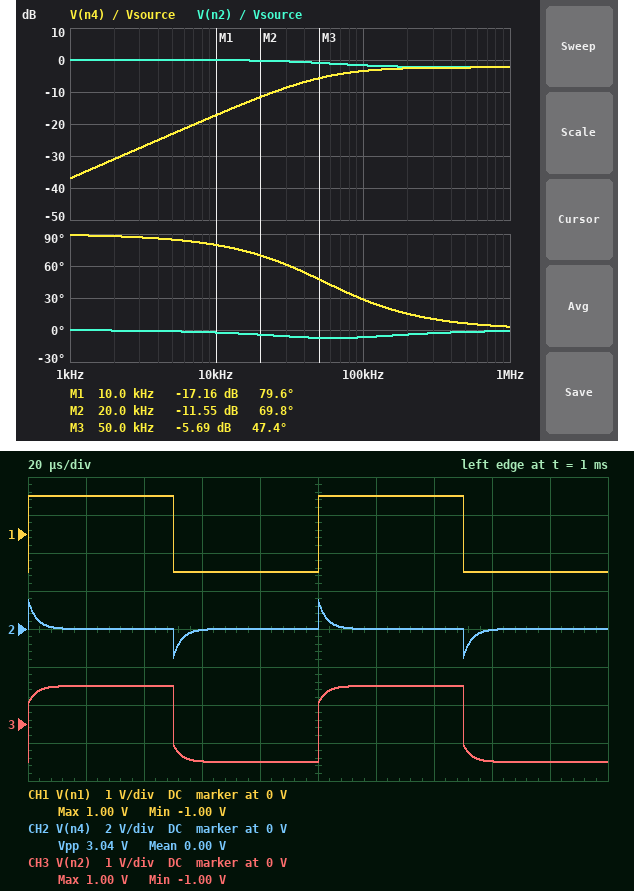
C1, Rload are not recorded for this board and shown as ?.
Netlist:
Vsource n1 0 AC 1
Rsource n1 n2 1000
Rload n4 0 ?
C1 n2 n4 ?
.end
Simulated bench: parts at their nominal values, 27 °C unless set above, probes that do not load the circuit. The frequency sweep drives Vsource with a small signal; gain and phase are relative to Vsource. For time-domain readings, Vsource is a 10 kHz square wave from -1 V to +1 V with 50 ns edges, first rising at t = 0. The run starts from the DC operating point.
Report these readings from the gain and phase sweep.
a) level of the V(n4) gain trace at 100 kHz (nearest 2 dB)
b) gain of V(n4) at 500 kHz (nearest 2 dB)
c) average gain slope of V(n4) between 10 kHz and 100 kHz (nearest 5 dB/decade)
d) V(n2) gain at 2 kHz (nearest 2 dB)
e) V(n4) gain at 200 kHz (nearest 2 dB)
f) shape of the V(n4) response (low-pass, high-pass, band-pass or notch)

-4 dB
-2 dB
15 dB/decade
0 dB
-2 dB
high-pass
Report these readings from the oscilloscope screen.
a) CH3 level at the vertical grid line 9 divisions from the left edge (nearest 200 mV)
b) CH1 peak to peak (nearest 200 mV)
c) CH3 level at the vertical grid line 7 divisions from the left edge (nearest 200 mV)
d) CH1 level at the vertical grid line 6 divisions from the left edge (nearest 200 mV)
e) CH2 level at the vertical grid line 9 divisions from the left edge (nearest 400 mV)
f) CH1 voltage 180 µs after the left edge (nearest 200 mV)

-1.0 V
2.0 V
1.0 V
1.0 V
0 V
-1.0 V
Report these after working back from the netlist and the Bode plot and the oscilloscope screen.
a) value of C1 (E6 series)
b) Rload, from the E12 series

680 pF
3.3 kΩ
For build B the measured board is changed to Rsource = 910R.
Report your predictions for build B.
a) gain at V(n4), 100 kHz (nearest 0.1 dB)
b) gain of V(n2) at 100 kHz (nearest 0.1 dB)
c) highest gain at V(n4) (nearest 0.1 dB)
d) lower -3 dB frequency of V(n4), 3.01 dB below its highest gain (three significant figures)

-3.3 dB
-1.5 dB
-2.1 dB
55.6 kHz
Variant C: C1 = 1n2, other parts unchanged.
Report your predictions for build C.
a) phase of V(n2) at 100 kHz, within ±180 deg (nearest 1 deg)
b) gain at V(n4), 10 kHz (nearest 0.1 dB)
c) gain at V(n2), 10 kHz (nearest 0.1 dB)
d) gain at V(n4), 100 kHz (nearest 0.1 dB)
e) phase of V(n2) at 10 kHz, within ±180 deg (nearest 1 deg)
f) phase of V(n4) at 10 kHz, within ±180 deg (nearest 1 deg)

-5 deg
-12.5 dB
-0.2 dB
-2.7 dB
-4 deg
72 deg
